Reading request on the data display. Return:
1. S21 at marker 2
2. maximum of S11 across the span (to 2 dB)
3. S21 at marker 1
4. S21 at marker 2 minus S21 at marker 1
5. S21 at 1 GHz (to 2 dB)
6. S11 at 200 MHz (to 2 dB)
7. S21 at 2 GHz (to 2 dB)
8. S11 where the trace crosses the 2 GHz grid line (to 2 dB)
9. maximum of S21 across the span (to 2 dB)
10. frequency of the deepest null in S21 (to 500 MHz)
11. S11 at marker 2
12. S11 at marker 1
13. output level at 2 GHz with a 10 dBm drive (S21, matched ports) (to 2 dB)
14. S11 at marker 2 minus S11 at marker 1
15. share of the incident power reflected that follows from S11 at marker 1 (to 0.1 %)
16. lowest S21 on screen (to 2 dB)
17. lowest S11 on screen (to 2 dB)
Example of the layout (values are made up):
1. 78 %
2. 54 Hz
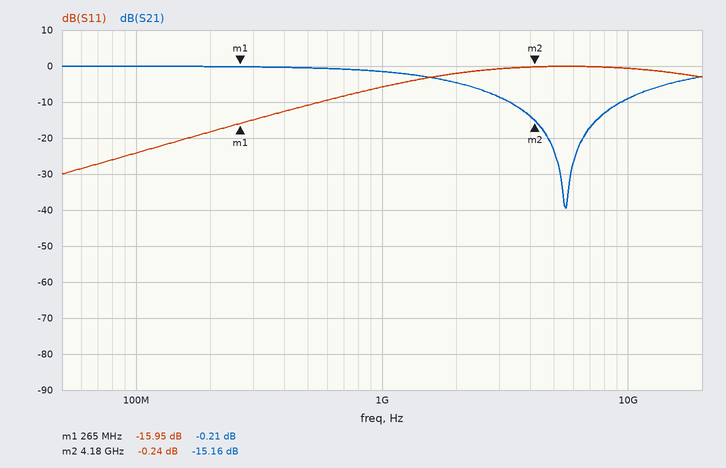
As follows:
1. -15.16 dB
2. 0 dB
3. -0.21 dB
4. -14.95 dB
5. -2 dB
6. -18 dB
7. -4 dB
8. -2 dB
9. 0 dB
10. 5.5 GHz
11. -0.24 dB
12. -15.95 dB
13. 6 dBm
14. 15.71 dB
15. 2.5 %
16. -40 dB
17. -30 dB
